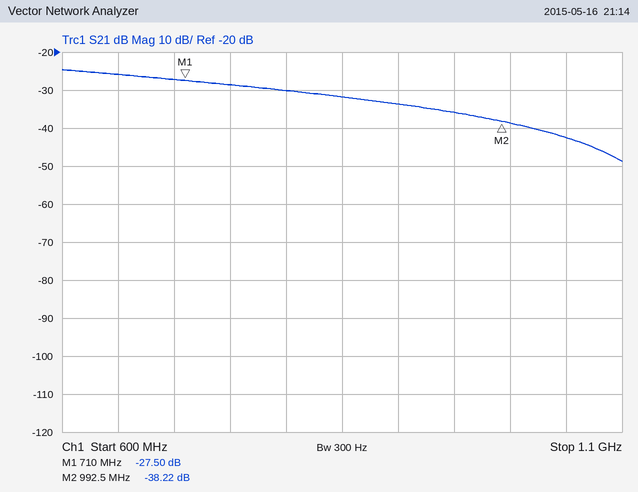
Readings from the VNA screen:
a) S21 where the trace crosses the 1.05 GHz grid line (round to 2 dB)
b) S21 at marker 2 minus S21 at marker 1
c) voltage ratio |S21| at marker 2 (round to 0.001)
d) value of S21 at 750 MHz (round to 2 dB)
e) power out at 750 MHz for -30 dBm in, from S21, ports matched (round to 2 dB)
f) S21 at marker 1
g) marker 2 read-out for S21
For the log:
-42 dB
-10.72 dB
0.012
-28 dB
-58 dBm
-27.50 dB
-38.22 dB
